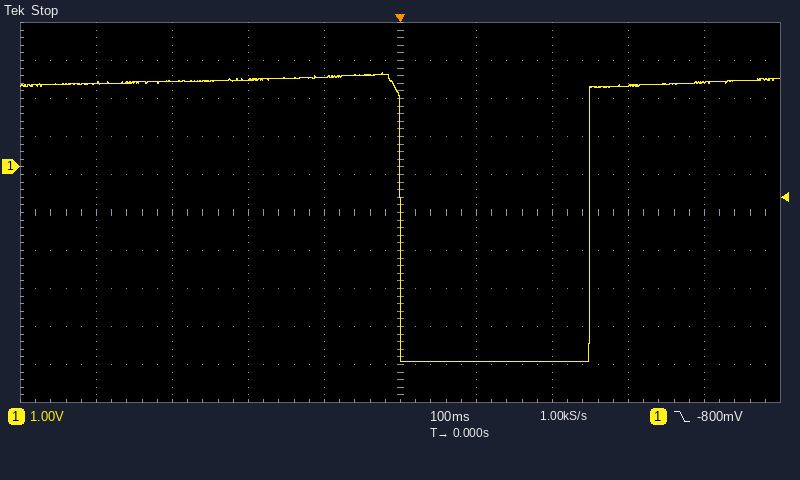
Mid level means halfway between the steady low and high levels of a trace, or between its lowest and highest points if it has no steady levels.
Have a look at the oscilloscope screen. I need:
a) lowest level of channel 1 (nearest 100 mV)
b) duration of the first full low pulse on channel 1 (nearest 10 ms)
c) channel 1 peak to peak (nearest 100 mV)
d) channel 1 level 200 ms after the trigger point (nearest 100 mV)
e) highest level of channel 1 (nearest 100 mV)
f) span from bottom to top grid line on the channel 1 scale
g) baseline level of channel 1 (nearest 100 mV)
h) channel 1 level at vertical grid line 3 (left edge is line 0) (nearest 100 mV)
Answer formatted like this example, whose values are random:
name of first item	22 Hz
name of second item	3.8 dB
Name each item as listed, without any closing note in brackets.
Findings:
lowest level of channel 1	-5.1 V
duration of the first full low pulse on channel 1	250 ms
channel 1 peak to peak	7.6 V
channel 1 level 200 ms after the trigger point	-5.1 V
highest level of channel 1	2.5 V
span from bottom to top grid line on the channel 1 scale	10 V
baseline level of channel 1	2.2 V
channel 1 level at vertical grid line 3 (left edge is line 0)	2.3 V
